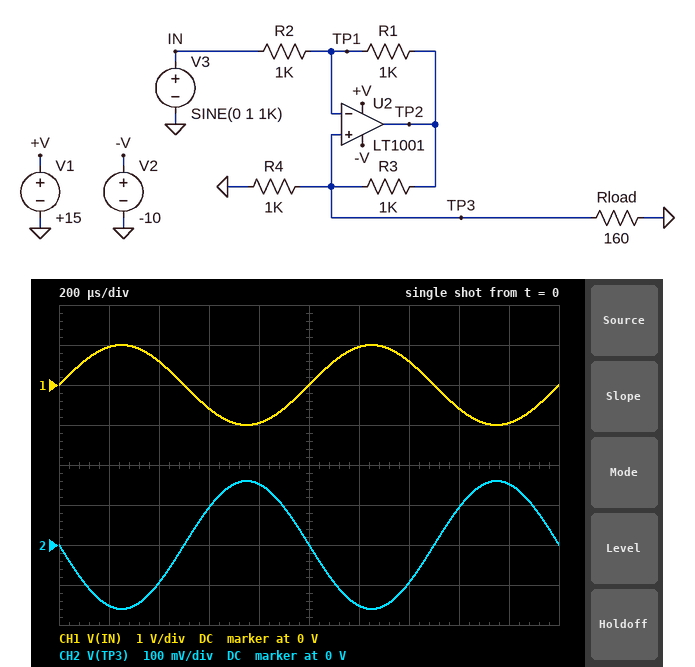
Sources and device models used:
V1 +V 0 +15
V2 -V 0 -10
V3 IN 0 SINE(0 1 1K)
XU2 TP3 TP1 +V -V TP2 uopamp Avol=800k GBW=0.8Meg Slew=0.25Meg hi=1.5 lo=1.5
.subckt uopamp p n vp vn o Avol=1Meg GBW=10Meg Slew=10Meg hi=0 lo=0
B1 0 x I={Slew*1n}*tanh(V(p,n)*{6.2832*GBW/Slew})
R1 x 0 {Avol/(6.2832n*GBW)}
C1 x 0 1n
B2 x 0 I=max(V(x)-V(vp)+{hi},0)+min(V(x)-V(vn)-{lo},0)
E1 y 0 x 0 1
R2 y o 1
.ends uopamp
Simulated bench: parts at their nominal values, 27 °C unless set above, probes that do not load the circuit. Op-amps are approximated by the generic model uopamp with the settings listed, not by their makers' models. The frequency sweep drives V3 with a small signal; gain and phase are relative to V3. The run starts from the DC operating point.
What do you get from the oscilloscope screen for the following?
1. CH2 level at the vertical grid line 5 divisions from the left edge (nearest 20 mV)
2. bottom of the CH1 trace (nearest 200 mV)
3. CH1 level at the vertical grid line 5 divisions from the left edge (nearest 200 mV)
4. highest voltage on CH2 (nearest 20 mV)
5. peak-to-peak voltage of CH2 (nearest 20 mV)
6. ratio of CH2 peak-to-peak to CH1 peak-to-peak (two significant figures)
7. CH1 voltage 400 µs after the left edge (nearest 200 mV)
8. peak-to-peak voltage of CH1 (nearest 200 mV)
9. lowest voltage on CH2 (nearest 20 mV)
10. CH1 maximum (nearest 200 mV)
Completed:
0 V
-1.0 V
0 V
160 mV
320 mV
0.16
600 mV
2.0 V
-160 mV
1.0 V
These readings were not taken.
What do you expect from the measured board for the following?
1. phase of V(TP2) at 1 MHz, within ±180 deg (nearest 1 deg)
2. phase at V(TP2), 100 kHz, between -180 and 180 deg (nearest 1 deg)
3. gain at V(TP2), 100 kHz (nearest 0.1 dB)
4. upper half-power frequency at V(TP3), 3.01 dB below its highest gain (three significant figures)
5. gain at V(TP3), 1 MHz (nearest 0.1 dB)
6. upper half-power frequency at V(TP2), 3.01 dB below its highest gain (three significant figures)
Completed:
107 deg
162 deg
2.0 dB
303 kHz
-26.7 dB
303 kHz
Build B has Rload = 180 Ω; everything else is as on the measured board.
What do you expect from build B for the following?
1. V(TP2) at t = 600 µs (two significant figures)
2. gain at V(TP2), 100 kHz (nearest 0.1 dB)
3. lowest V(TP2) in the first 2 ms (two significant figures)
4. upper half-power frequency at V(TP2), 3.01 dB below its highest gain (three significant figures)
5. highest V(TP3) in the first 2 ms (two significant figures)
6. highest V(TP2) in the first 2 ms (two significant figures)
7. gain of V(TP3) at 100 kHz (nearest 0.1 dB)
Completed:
800 mV
2.2 dB
-1.4 V
294 kHz
180 mV
1.4 V
-15.4 dB
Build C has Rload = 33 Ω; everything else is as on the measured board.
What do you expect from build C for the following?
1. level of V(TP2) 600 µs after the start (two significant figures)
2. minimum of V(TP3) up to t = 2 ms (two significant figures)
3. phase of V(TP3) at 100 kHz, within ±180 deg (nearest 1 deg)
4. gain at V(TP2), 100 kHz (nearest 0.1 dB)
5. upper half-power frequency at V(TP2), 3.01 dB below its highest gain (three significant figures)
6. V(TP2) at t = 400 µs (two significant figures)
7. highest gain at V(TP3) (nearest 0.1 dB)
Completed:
620 mV
-33 mV
165 deg
0.3 dB
375 kHz
-630 mV
-29.6 dB
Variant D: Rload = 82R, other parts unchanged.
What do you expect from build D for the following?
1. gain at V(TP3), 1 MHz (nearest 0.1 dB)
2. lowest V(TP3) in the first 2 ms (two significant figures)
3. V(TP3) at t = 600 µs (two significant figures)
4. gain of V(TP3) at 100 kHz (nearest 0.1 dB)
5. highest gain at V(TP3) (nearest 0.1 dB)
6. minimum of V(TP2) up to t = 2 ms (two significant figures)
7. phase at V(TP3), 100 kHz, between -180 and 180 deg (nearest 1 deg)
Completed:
-31.5 dB
-82 mV
48 mV
-22.1 dB
-21.7 dB
-1.2 V
164 deg
